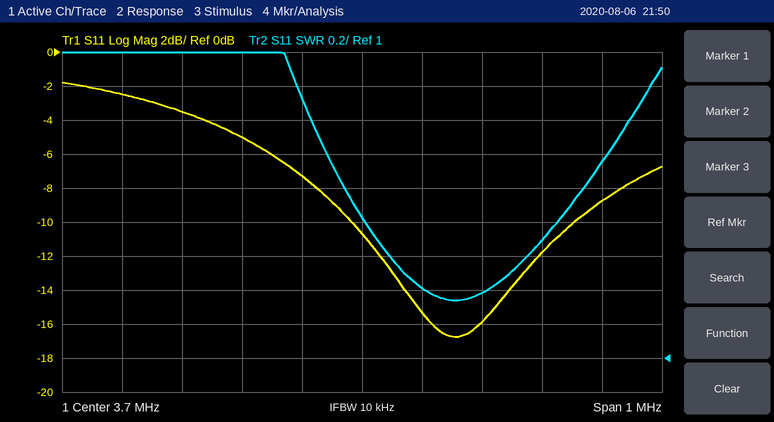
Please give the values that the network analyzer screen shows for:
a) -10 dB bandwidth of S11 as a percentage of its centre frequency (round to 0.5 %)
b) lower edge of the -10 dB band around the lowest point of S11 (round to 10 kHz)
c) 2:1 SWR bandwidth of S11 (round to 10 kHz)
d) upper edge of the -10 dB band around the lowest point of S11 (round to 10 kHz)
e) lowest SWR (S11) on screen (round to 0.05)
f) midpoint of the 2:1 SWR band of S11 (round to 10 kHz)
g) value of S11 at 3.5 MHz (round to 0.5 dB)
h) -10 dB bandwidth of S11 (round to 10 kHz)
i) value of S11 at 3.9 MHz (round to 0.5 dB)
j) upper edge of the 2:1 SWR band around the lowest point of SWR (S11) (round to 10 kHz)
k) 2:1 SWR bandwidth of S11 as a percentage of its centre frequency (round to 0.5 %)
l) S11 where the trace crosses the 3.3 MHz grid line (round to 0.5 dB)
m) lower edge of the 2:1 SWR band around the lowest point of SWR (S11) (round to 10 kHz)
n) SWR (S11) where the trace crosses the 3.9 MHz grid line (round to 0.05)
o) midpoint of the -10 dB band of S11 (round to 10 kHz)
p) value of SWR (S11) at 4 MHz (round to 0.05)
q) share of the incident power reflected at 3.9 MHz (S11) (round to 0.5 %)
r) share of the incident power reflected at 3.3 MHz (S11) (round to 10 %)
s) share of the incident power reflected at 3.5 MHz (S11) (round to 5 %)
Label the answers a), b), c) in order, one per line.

a) 9.5 %
b) 3.68 MHz
c) 400 kHz
d) 4.05 MHz
e) 1.35
f) 3.87 MHz
g) -5.0 dB
h) 370 kHz
i) -16.0 dB
j) 4.07 MHz
k) 10.5 %
l) -2.5 dB
m) 3.67 MHz
n) 1.40
o) 3.87 MHz
p) 1.70
q) 2.5 %
r) 60 %
s) 30 %
